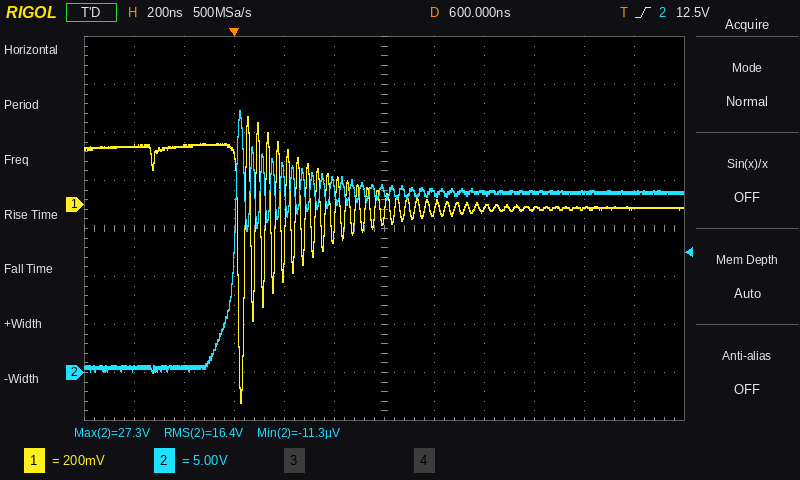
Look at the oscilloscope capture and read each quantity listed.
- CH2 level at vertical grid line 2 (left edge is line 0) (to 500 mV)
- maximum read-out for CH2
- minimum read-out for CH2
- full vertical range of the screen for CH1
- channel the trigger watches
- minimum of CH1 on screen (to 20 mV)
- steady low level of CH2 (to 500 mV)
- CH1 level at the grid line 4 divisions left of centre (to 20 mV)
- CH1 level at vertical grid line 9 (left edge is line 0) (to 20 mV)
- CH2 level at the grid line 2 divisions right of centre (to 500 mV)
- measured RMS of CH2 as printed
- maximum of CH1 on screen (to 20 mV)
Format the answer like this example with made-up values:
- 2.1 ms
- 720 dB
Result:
- 500 mV
- 27.3 V
- -11.3 µV
- 1.6 V
- CH2
- -820 mV
- 500 mV
- 240 mV
- -20 mV
- 18.5 V
- 16.4 V
- 360 mV
